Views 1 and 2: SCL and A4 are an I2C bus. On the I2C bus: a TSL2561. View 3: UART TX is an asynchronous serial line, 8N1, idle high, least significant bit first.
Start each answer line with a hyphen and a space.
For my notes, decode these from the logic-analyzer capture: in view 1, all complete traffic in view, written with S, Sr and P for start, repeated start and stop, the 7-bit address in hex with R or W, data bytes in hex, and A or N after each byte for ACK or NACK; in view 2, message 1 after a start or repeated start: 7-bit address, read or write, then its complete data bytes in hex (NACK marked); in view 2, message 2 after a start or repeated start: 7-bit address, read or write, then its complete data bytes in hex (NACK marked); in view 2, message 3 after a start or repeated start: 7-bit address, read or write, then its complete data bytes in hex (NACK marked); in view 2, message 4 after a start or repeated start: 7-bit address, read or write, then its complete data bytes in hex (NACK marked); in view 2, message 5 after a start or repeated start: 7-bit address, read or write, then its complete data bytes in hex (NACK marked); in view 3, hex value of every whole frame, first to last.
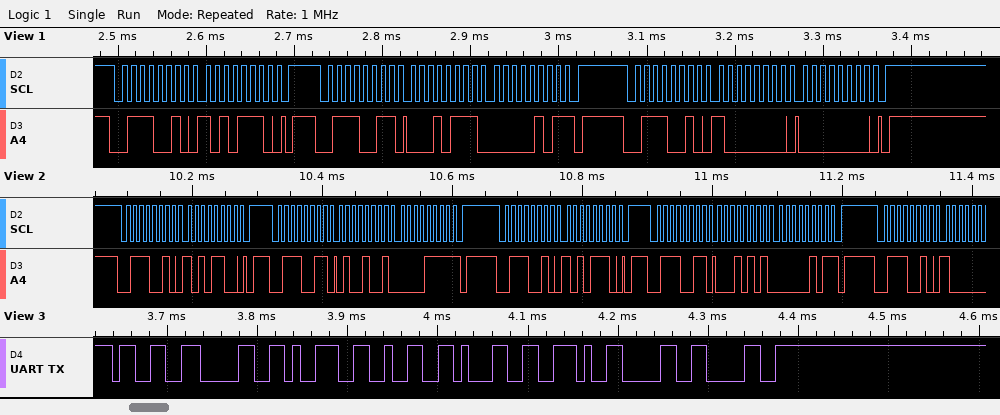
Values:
- S 39W A AE A P S 39R A 17 A 05 N P S 39W A 80 A 00 A P
- 0x39 write: AC
- 0x39 read: 49 0F NACK
- 0x39 write: AE
- 0x39 read: 15 05 NACK
- 0x39 write
- 33 30 39 32 31 2E 30 30
